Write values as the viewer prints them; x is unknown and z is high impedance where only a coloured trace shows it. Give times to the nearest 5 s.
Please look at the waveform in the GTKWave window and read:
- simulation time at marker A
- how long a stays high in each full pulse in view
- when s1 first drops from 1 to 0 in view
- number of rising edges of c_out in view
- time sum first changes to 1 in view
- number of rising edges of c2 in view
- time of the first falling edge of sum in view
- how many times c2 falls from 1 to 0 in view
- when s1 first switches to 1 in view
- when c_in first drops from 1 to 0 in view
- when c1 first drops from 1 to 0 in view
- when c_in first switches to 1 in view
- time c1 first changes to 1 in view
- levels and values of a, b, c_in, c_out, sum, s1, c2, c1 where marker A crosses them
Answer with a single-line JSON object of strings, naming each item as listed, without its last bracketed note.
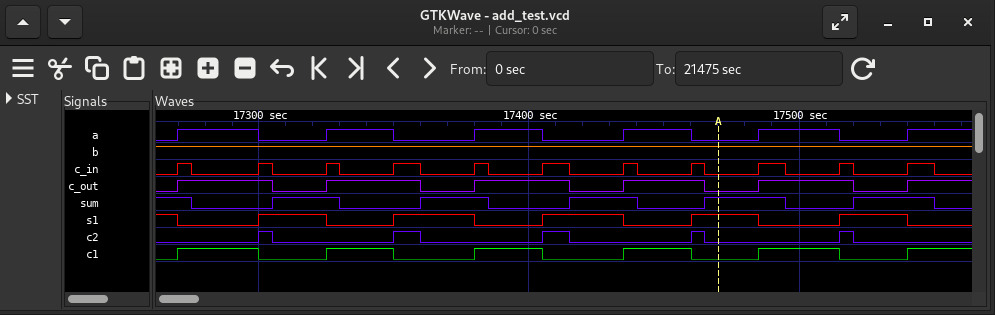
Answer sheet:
{"simulation time at marker A": "17470 s", "how long a stays high in each full pulse in view": "30 s, 25 s, 25 s, 25 s, 30 s", "when s1 first drops from 1 to 0 in view": "17270 s", "number of rising edges of c_out in view": "6", "time sum first changes to 1 in view": "17305 s", "number of rising edges of c2 in view": "5", "time of the first falling edge of sum in view": "17275 s", "how many times c2 falls from 1 to 0 in view": "5", "when s1 first switches to 1 in view": "17300 s", "when c_in first drops from 1 to 0 in view": "17275 s", "when c1 first drops from 1 to 0 in view": "17300 s", "when c_in first switches to 1 in view": "17270 s", "time c1 first changes to 1 in view": "17270 s", "levels and values of a, b, c_in, c_out, sum, s1, c2, c1 where marker A crosses them": "a=0, b=1, c_in=0, c_out=0, sum=1, s1=1, c2=0, c1=0"}
